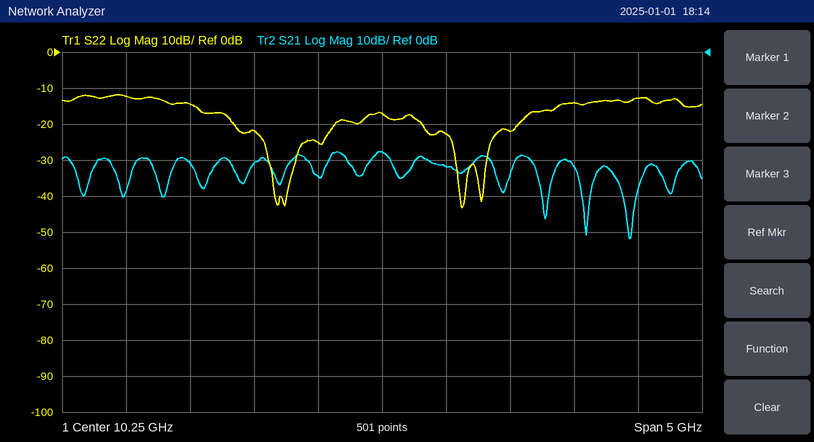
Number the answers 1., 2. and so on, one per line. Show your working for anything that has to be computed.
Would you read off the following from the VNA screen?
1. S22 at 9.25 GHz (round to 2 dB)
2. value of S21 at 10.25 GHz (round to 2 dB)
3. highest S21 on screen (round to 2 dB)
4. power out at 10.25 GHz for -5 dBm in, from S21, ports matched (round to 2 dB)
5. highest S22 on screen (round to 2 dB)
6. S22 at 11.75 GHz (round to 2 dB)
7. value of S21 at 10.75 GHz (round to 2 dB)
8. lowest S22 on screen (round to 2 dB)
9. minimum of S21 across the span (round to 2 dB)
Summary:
1. -22 dB
2. -28 dB
3. -28 dB
4. -5 dBm + (-28 dB) = -32 dBm
5. -12 dB
6. -14 dB
7. -32 dB
8. -44 dB
9. -52 dB
